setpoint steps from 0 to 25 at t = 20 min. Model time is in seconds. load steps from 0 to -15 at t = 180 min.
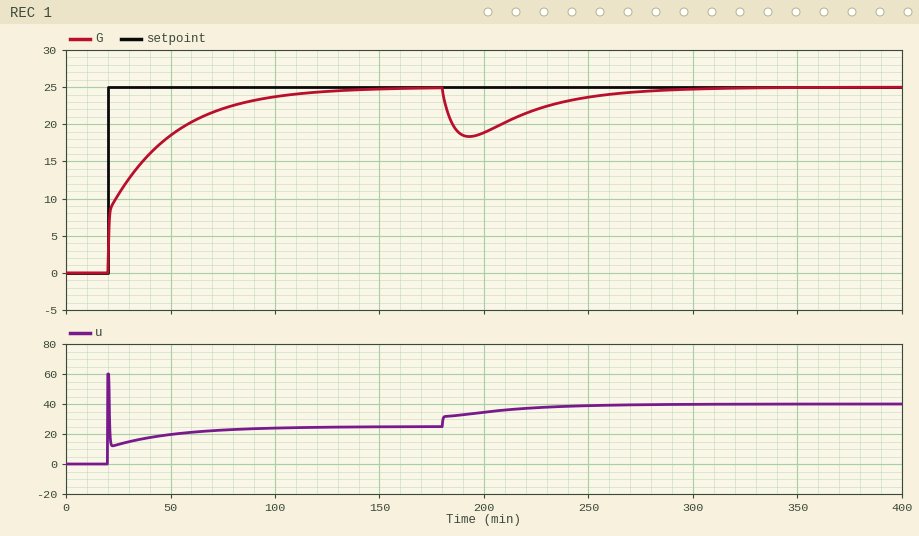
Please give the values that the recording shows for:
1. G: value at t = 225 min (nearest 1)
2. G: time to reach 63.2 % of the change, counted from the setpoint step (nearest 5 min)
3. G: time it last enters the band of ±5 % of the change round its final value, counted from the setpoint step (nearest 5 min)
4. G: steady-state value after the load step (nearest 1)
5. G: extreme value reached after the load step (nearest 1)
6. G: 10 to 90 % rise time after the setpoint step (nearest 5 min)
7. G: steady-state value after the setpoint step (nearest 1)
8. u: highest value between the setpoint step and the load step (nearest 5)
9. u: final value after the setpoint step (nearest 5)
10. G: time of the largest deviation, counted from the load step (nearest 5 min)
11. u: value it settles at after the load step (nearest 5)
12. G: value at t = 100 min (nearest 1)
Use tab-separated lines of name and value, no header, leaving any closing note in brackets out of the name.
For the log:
G: value at t = 225 min	22
G: time to reach 63.2 % of the change, counted from the setpoint step	20 min
G: time it last enters the band of ±5 % of the change round its final value, counted from the setpoint step	80 min
G: steady-state value after the load step	25
G: extreme value reached after the load step	18
G: 10 to 90 % rise time after the setpoint step	60 min
G: steady-state value after the setpoint step	25
u: highest value between the setpoint step and the load step	60
u: final value after the setpoint step	25
G: time of the largest deviation, counted from the load step	15 min
u: value it settles at after the load step	40
G: value at t = 100 min	24
